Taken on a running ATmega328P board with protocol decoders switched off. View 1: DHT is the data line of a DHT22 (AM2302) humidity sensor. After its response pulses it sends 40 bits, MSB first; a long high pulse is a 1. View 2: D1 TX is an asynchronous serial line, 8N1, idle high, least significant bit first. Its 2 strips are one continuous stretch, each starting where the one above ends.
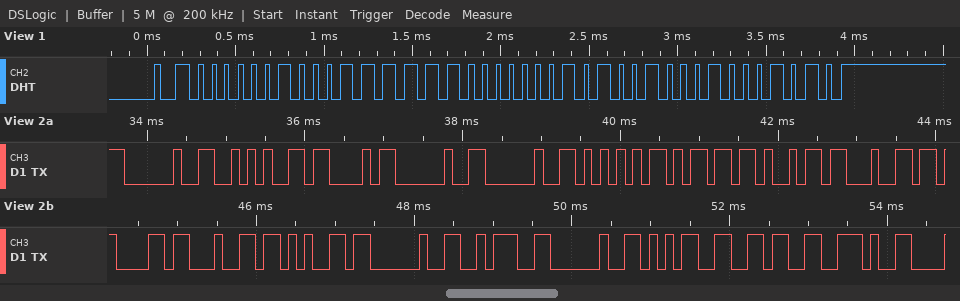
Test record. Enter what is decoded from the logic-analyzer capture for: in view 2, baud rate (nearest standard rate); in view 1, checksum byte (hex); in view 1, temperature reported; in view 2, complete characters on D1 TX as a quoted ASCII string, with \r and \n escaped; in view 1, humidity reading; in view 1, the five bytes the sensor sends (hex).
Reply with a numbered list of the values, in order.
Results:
1. 9600 baud
2. 0x8A
3. 32.8 °C
4. " *C  Umidade : 56."
5. 57.5 %
6. 02 3F 01 48 8A
